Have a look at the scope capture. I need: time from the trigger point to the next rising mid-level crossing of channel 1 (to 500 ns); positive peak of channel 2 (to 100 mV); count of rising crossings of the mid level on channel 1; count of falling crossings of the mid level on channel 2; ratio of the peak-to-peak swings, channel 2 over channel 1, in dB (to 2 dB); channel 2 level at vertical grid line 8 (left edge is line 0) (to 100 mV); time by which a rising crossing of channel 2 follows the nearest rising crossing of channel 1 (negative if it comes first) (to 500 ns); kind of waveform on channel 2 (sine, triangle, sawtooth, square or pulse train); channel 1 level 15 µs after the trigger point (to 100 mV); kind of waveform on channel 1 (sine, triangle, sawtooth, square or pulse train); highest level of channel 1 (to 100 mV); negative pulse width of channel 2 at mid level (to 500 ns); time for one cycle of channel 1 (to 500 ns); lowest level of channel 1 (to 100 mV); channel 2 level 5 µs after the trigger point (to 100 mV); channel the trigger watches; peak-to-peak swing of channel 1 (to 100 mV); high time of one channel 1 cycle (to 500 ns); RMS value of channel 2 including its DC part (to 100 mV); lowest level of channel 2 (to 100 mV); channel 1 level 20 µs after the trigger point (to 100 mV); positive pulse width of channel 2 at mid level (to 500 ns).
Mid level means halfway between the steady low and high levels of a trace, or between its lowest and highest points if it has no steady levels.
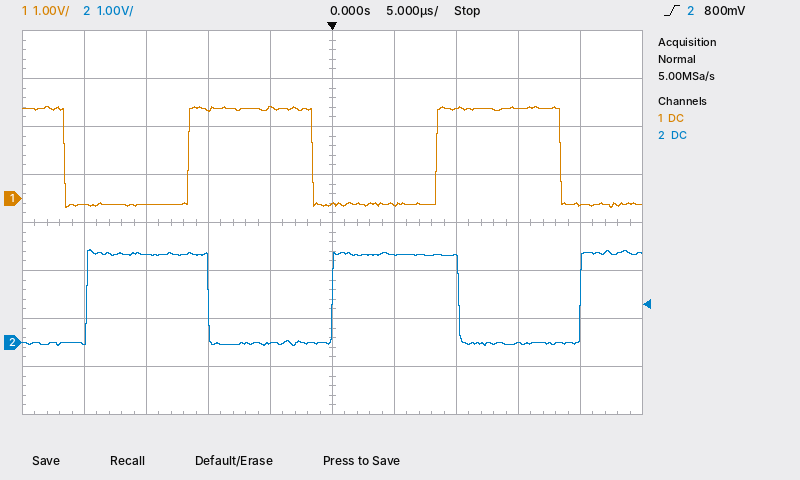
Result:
8.5 µs
1.9 V
2
2
0 dB
0.0 V
-8.5 µs
square
1.9 V
square
1.9 V
10.0 µs
20.0 µs
-200 mV
1.8 V
channel 2
2.1 V
10.0 µs
1.3 V
-100 mV
-100 mV
10.0 µs
